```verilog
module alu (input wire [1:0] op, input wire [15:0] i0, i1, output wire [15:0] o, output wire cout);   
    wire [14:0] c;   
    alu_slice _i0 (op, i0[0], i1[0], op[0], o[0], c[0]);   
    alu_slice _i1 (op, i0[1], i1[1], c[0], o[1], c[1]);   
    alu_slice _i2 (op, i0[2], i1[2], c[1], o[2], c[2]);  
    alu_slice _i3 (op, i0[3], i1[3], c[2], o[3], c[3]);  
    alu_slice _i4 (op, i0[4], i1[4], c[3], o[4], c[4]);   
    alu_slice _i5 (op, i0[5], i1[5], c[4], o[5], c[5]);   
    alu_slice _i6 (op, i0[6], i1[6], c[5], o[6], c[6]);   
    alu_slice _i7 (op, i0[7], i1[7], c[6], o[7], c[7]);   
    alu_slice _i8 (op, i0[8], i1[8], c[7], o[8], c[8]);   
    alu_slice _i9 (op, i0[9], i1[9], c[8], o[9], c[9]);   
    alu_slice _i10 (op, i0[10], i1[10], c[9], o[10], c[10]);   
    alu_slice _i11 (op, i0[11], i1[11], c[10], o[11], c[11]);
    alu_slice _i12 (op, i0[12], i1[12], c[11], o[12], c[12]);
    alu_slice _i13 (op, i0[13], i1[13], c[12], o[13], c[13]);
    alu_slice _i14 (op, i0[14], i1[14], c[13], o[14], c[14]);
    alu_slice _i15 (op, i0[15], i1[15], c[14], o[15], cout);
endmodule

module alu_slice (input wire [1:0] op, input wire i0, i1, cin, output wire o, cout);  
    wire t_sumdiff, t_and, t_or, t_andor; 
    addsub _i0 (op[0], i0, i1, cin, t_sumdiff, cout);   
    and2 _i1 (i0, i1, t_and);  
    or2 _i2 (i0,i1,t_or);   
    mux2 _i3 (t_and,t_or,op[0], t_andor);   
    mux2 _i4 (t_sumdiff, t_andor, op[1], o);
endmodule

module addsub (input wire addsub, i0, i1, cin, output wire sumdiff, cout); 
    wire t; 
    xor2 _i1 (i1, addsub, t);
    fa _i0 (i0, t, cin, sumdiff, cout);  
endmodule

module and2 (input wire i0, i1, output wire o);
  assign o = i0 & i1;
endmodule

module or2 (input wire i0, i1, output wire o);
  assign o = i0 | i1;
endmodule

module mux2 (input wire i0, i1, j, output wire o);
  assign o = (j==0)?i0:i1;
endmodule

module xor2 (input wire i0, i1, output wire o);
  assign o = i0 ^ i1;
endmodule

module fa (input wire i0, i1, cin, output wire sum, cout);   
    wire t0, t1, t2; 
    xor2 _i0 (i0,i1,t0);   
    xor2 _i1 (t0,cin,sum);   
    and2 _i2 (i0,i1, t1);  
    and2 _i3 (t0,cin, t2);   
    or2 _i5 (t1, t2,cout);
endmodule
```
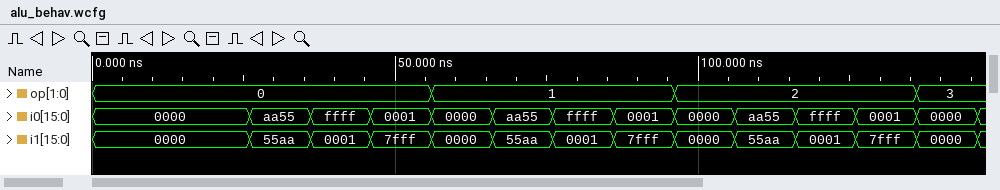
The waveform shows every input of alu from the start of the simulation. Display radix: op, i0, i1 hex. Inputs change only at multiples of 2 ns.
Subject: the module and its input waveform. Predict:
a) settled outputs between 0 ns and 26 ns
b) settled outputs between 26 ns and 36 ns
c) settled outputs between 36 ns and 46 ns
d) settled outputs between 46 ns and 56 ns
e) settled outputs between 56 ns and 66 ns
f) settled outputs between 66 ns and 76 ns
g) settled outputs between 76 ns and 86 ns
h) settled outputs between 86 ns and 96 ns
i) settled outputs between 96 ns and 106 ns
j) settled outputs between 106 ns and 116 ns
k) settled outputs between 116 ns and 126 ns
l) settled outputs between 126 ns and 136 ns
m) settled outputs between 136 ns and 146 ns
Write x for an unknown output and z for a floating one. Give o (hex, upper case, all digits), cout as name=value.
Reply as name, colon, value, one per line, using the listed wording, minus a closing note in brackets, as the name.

settled outputs between 0 ns and 26 ns: o=0000, cout=0
settled outputs between 26 ns and 36 ns: o=FFFF, cout=0
settled outputs between 36 ns and 46 ns: o=0000, cout=1
settled outputs between 46 ns and 56 ns: o=8000, cout=0
settled outputs between 56 ns and 66 ns: o=0000, cout=1
settled outputs between 66 ns and 76 ns: o=54AB, cout=1
settled outputs between 76 ns and 86 ns: o=FFFE, cout=1
settled outputs between 86 ns and 96 ns: o=8002, cout=0
settled outputs between 96 ns and 106 ns: o=0000, cout=0
settled outputs between 106 ns and 116 ns: o=0000, cout=0
settled outputs between 116 ns and 126 ns: o=0001, cout=1
settled outputs between 126 ns and 136 ns: o=0001, cout=0
settled outputs between 136 ns and 146 ns: o=0000, cout=1
